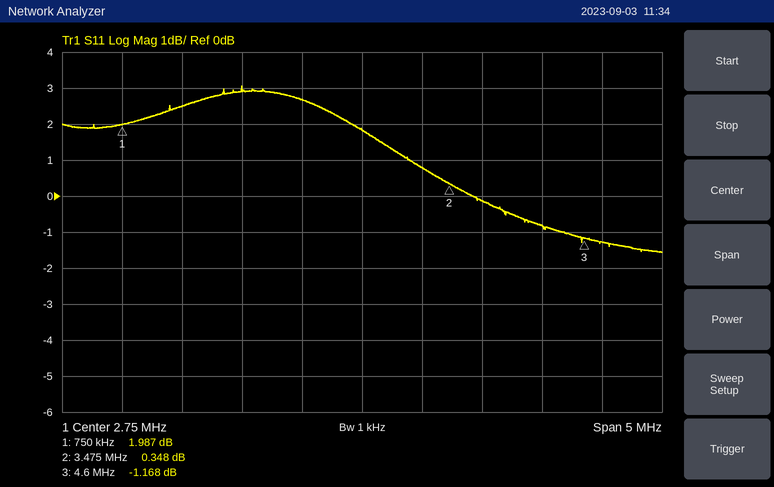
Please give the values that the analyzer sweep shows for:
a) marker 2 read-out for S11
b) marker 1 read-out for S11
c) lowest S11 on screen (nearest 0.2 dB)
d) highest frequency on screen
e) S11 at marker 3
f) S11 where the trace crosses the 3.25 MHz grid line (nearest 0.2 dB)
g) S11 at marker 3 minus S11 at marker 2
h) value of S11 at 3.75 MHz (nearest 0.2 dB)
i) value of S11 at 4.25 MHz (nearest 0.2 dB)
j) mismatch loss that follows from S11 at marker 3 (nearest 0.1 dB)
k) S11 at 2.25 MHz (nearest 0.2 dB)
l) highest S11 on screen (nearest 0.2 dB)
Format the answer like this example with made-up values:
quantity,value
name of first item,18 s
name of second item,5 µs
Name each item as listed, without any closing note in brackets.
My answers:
quantity,value
marker 2 read-out for S11,0.348 dB
marker 1 read-out for S11,1.987 dB
lowest S11 on screen,-1.6 dB
highest frequency on screen,5.25 MHz
S11 at marker 3,-1.168 dB
S11 where the trace crosses the 3.25 MHz grid line,0.8 dB
S11 at marker 3 minus S11 at marker 2,-1.516 dB
value of S11 at 3.75 MHz,-0.2 dB
value of S11 at 4.25 MHz,-0.8 dB
mismatch loss that follows from S11 at marker 3,6.3 dB
S11 at 2.25 MHz,2.6 dB
highest S11 on screen,3.0 dB
